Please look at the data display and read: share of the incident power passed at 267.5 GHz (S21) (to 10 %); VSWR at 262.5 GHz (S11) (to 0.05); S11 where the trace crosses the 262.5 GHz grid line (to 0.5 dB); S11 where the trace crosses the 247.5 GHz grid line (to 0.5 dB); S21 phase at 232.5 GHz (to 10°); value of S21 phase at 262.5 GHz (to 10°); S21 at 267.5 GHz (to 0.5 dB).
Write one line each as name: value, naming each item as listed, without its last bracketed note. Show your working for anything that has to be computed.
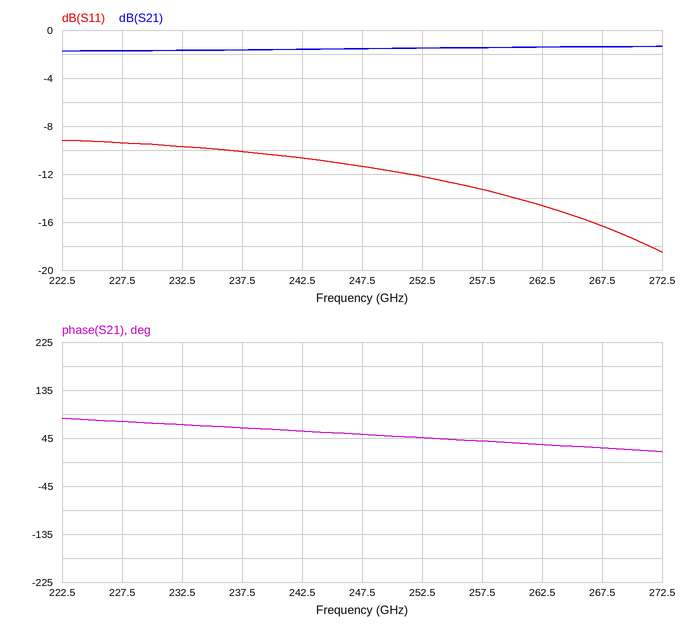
share of the incident power passed at 267.5 GHz (S21): 10^(-1.5/10) ≈ 70.8 %, so 70 % to the nearest 10 %
VSWR at 262.5 GHz (S11): |Γ| = 10^(-14.5/20) = 0.1884; VSWR = (1 + 0.1884)/(1 − 0.1884) ≈ 1.46, so 1.45 to the nearest 0.05
S11 where the trace crosses the 262.5 GHz grid line: -14.5 dB
S11 where the trace crosses the 247.5 GHz grid line: -11.5 dB
S21 phase at 232.5 GHz: 70°
value of S21 phase at 262.5 GHz: 30°
S21 at 267.5 GHz: -1.5 dB
